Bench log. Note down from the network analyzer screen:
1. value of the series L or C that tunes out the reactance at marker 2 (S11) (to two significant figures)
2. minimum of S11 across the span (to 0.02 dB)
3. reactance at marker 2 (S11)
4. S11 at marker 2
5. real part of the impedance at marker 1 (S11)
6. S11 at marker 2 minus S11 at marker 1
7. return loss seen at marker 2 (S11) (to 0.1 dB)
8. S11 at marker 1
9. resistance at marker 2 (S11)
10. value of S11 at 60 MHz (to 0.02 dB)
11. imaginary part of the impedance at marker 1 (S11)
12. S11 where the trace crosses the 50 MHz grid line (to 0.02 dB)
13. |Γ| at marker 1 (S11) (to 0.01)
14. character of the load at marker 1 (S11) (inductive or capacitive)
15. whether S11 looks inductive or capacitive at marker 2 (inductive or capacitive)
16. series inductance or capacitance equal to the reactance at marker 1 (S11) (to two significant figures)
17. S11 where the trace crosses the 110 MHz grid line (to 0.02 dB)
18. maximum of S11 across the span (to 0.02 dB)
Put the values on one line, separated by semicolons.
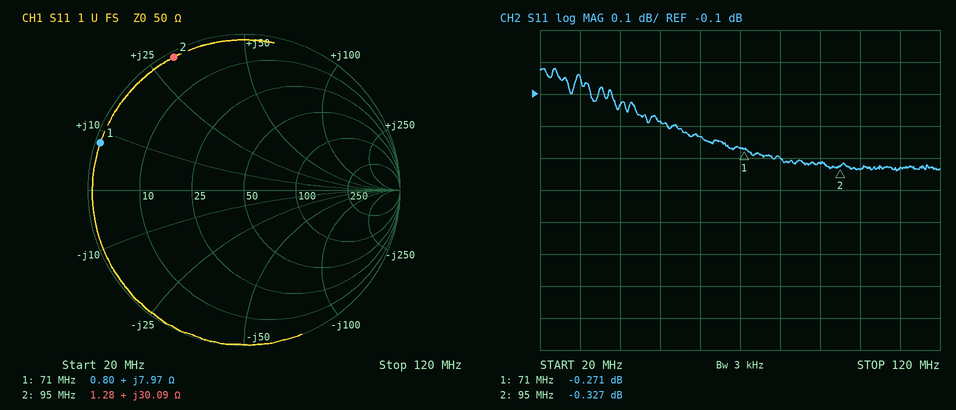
56 pF; -0.34 dB; +30.09 Ω; -0.327 dB; 0.80 Ω; -0.056 dB; 0.3 dB; -0.271 dB; 1.28 Ω; -0.24 dB; +7.97 Ω; -0.18 dB; 0.97; inductive; inductive; 18 nH; -0.34 dB; -0.02 dB
